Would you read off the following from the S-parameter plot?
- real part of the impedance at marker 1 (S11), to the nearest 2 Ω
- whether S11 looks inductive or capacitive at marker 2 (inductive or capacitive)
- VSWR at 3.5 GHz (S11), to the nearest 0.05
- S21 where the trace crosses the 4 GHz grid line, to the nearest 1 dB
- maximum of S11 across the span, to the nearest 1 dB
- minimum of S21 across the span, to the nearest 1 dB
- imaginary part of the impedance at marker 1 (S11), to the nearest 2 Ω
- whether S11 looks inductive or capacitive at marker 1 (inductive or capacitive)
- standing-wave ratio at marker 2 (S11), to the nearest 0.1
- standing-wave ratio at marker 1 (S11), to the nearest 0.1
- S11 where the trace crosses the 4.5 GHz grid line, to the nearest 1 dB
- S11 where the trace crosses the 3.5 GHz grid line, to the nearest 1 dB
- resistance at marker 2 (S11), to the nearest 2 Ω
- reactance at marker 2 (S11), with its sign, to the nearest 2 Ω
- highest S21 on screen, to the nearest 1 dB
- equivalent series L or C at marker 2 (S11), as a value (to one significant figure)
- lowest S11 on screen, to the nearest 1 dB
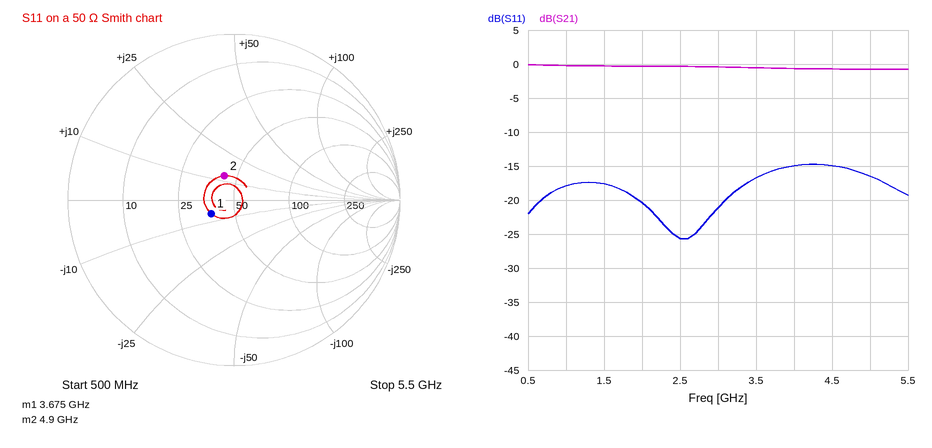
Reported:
38 Ω
inductive
1.35
-1 dB
-15 dB
-1 dB
-6 Ω
capacitive
1.4
1.4
-15 dB
-17 dB
42 Ω
+12 Ω
0 dB
400 pH
-26 dB
